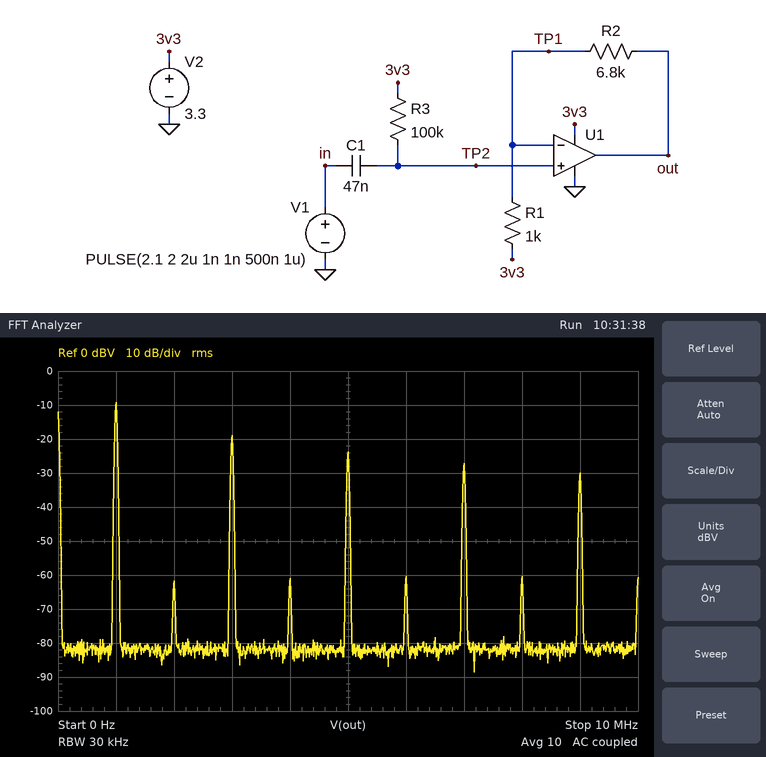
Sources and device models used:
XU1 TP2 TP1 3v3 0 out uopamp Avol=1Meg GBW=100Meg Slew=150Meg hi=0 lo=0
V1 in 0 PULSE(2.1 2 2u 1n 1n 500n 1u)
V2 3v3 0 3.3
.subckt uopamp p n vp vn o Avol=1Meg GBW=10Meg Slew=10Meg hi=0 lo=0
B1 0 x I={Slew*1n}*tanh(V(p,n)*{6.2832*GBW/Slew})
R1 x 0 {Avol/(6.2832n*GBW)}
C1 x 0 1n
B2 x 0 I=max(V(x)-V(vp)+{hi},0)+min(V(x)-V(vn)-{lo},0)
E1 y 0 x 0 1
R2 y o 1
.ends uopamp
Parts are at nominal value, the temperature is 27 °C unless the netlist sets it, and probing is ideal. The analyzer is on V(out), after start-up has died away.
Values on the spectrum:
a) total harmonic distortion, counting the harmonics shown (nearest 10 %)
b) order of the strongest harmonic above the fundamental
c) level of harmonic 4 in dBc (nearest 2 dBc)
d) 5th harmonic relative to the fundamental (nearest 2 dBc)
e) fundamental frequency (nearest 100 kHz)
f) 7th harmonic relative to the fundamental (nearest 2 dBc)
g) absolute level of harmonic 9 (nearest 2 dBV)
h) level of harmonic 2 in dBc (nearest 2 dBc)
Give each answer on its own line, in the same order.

40 %
3
-52 dBc
-14 dBc
1.0 MHz
-18 dBc
-30 dBV
-52 dBc
